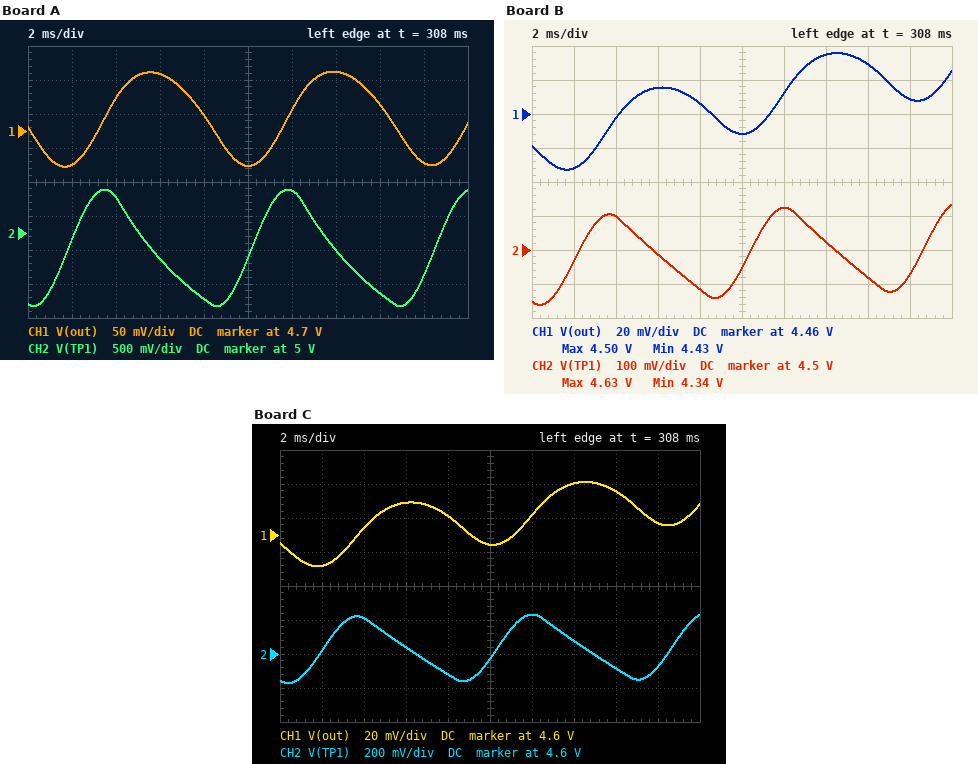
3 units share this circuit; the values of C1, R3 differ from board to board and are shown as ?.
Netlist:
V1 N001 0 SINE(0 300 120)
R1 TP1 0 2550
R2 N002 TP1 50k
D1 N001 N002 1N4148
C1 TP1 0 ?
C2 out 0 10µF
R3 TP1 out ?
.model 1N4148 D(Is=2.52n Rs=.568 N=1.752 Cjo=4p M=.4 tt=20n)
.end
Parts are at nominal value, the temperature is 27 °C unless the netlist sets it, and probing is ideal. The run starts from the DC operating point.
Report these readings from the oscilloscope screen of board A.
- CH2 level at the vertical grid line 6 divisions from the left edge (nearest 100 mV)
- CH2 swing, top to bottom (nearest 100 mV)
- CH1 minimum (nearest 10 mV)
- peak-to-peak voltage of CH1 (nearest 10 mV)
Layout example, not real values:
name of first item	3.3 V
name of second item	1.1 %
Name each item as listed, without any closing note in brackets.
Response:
CH2 level at the vertical grid line 6 divisions from the left edge	5.6 V
CH2 swing, top to bottom	1.7 V
CH1 minimum	4.65 V
peak-to-peak voltage of CH1	140 mV
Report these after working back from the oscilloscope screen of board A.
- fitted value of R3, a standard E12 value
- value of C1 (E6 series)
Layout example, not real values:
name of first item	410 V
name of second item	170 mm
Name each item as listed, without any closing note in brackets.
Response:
fitted value of R3, a standard E12 value	1.5 kΩ
value of C1	4.7 µF
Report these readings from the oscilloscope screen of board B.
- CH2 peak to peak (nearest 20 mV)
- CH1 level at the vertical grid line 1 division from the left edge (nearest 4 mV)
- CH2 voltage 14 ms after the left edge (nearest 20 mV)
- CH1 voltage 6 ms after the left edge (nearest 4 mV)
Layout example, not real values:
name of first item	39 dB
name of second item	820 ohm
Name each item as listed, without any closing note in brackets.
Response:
CH2 peak to peak	300 mV
CH1 level at the vertical grid line 1 division from the left edge	4.428 V
CH2 voltage 14 ms after the left edge	4.52 V
CH1 voltage 6 ms after the left edge	4.476 V
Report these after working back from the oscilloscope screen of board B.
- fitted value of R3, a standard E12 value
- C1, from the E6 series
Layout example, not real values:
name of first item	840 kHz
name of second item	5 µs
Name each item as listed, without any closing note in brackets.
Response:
fitted value of R3, a standard E12 value	820 Ω
C1, from the E6 series	33 µF
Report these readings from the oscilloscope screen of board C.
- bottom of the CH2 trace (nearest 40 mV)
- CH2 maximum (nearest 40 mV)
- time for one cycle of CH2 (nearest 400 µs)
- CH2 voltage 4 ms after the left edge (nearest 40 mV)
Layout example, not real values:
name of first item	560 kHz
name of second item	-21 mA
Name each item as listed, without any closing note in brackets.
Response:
bottom of the CH2 trace	4.44 V
CH2 maximum	4.84 V
time for one cycle of CH2	8.4 ms
CH2 voltage 4 ms after the left edge	4.80 V
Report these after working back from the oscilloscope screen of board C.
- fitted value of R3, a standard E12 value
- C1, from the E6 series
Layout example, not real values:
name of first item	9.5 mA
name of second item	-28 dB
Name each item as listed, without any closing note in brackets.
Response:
fitted value of R3, a standard E12 value	1.5 kΩ
C1, from the E6 series	22 µF
